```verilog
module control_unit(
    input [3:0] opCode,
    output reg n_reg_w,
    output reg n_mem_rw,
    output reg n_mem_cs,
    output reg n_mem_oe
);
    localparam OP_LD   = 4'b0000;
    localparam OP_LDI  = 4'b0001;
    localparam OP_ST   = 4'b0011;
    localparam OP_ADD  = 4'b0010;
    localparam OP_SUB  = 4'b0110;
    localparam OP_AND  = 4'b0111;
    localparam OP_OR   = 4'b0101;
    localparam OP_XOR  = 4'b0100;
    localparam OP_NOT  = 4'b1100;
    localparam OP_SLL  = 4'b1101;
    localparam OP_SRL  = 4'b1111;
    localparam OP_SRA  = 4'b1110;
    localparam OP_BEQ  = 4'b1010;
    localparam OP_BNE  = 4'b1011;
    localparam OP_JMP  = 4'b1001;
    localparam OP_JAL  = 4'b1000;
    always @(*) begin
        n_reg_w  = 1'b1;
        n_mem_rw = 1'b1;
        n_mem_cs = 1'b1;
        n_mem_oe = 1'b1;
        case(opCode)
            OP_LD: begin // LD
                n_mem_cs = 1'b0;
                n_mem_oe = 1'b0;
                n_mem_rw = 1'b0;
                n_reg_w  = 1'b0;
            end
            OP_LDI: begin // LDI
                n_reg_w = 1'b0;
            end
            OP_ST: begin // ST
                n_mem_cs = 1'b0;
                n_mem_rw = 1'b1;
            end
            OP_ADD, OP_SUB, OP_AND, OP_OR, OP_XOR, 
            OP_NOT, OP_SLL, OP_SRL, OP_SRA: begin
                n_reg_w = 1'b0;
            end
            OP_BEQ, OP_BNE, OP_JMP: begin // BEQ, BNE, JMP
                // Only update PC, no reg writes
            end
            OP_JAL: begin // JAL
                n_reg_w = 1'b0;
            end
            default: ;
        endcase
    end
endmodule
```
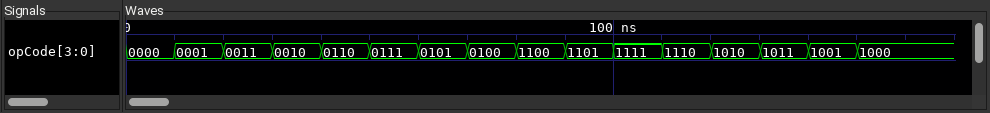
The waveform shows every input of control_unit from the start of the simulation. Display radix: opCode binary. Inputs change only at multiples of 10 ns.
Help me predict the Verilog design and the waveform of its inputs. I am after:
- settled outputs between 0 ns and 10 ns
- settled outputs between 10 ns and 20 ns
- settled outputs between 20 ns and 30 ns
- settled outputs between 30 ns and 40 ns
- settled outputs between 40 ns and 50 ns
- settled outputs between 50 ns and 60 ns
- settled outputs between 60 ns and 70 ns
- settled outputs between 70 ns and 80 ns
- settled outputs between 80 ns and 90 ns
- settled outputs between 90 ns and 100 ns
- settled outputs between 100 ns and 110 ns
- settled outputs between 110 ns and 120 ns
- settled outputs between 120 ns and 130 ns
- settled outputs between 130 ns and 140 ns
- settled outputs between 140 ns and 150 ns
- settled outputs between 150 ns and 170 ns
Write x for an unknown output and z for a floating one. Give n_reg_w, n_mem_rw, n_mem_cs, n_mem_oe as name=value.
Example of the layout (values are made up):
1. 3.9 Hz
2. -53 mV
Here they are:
1. n_reg_w=0, n_mem_rw=0, n_mem_cs=0, n_mem_oe=0
2. n_reg_w=0, n_mem_rw=1, n_mem_cs=1, n_mem_oe=1
3. n_reg_w=1, n_mem_rw=1, n_mem_cs=0, n_mem_oe=1
4. n_reg_w=0, n_mem_rw=1, n_mem_cs=1, n_mem_oe=1
5. n_reg_w=0, n_mem_rw=1, n_mem_cs=1, n_mem_oe=1
6. n_reg_w=0, n_mem_rw=1, n_mem_cs=1, n_mem_oe=1
7. n_reg_w=0, n_mem_rw=1, n_mem_cs=1, n_mem_oe=1
8. n_reg_w=0, n_mem_rw=1, n_mem_cs=1, n_mem_oe=1
9. n_reg_w=0, n_mem_rw=1, n_mem_cs=1, n_mem_oe=1
10. n_reg_w=0, n_mem_rw=1, n_mem_cs=1, n_mem_oe=1
11. n_reg_w=0, n_mem_rw=1, n_mem_cs=1, n_mem_oe=1
12. n_reg_w=0, n_mem_rw=1, n_mem_cs=1, n_mem_oe=1
13. n_reg_w=1, n_mem_rw=1, n_mem_cs=1, n_mem_oe=1
14. n_reg_w=1, n_mem_rw=1, n_mem_cs=1, n_mem_oe=1
15. n_reg_w=1, n_mem_rw=1, n_mem_cs=1, n_mem_oe=1
16. n_reg_w=0, n_mem_rw=1, n_mem_cs=1, n_mem_oe=1
